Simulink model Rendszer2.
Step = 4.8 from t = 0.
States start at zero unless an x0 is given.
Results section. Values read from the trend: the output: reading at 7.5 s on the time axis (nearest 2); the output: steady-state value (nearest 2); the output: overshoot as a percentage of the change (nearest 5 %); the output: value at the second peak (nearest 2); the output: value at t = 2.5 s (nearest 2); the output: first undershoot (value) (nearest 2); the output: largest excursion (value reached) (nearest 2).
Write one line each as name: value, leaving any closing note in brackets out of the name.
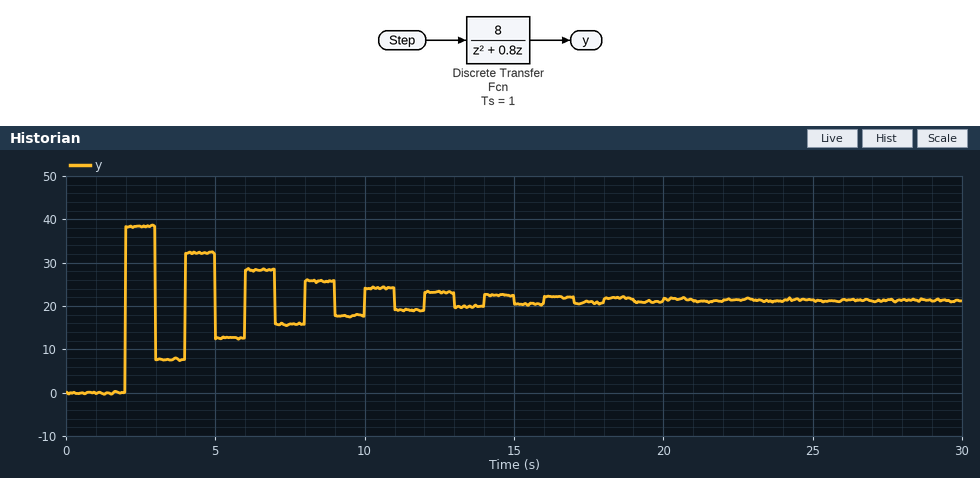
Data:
the output: reading at 7.5 s on the time axis: 16
the output: steady-state value: 22
the output: overshoot as a percentage of the change: 80 %
the output: value at the second peak: 32
the output: value at t = 2.5 s: 38
the output: first undershoot (value): 8
the output: largest excursion (value reached): 38
